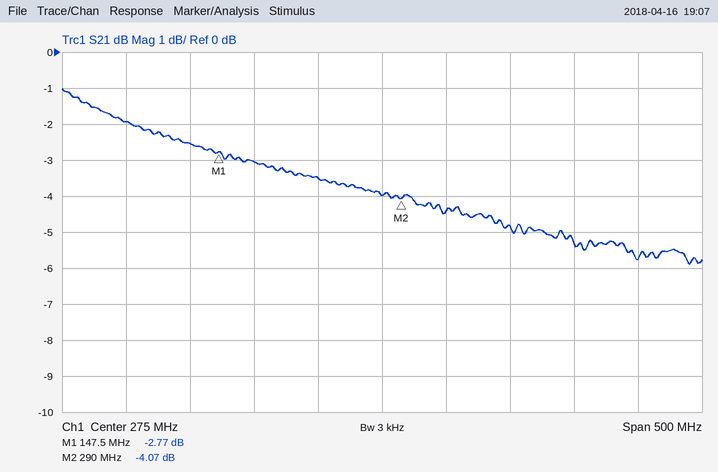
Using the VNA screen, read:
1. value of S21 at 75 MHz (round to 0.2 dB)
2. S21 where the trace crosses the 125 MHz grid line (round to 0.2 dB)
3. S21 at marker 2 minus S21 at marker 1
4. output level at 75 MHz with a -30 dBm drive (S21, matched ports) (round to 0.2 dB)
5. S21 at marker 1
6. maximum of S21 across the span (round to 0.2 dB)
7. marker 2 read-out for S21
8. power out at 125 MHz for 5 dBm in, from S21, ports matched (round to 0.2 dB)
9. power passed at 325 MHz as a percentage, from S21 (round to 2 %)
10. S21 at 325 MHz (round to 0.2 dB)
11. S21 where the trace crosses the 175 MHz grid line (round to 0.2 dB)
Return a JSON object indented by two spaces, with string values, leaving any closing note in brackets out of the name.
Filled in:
{
  "value of S21 at 75 MHz": "-2.0 dB",
  "S21 where the trace crosses the 125 MHz grid line": "-2.6 dB",
  "S21 at marker 2 minus S21 at marker 1": "-1.30 dB",
  "output level at 75 MHz with a -30 dBm drive (S21, matched ports)": "-32.0 dBm",
  "S21 at marker 1": "-2.77 dB",
  "maximum of S21 across the span": "-1.0 dB",
  "marker 2 read-out for S21": "-4.07 dB",
  "power out at 125 MHz for 5 dBm in, from S21, ports matched": "2.4 dBm",
  "power passed at 325 MHz as a percentage, from S21": "36 %",
  "S21 at 325 MHz": "-4.4 dB",
  "S21 where the trace crosses the 175 MHz grid line": "-3.0 dB"
}
